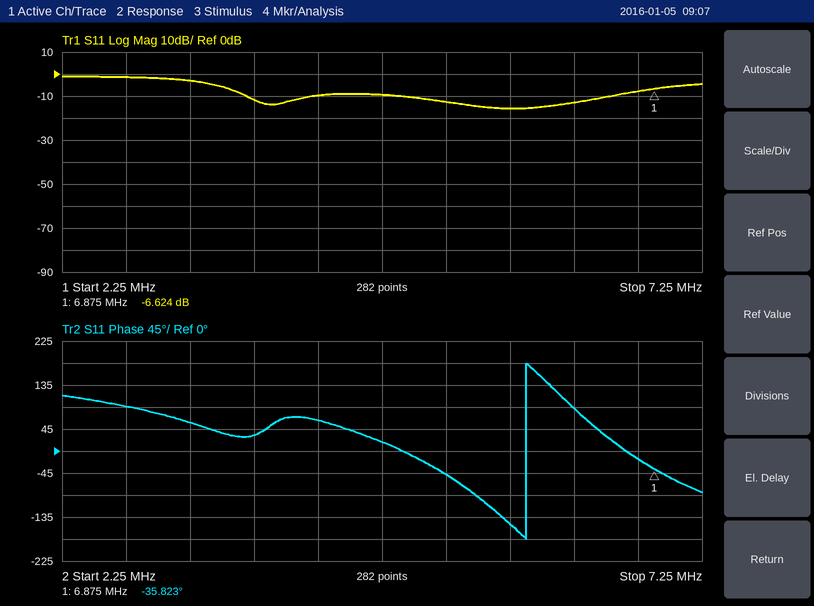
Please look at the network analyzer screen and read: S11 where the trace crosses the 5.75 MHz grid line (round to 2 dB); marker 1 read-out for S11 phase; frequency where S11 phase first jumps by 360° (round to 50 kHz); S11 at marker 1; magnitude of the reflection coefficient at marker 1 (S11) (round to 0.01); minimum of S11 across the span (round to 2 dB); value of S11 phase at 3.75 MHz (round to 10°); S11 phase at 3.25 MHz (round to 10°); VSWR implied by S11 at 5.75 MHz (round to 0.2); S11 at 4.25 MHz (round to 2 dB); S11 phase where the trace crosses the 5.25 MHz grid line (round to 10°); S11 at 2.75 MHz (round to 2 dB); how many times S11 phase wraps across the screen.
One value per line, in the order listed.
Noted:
-16 dB
-35.823°
5.90 MHz
-6.624 dB
0.47
-16 dB
30°
60°
1.4
-10 dB
-50°
-2 dB
1
